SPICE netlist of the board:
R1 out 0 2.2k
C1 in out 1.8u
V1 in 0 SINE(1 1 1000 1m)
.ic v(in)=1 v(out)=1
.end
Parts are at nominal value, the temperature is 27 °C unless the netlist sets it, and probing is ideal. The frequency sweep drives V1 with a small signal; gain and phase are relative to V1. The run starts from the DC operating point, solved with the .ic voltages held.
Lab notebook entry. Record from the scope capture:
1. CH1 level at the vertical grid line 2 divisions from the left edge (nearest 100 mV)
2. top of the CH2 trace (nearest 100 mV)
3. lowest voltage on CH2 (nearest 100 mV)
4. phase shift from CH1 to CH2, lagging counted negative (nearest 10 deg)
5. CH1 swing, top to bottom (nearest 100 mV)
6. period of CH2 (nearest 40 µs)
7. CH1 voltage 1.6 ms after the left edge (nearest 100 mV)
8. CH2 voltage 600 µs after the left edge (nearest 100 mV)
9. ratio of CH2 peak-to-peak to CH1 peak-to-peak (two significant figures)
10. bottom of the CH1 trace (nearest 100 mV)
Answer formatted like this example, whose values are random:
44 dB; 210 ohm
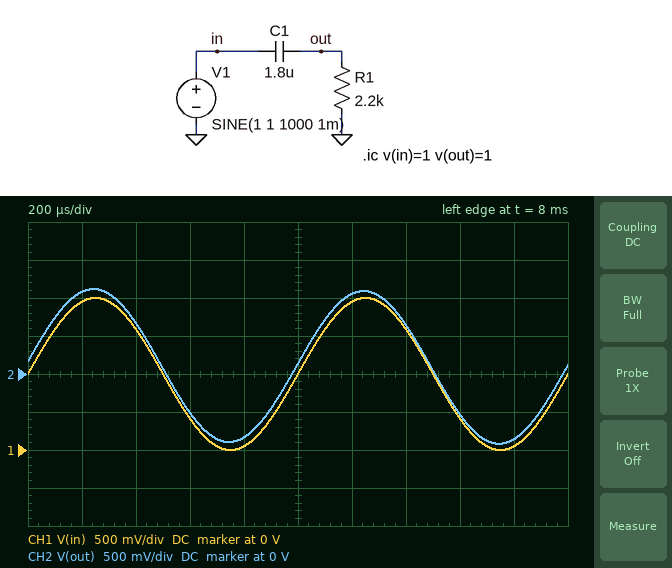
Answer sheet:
1.6 V; 1.1 V; -900 mV; 0 deg; 2.0 V; 1.00 ms; 400 mV; -500 mV; 1.0; 0 V
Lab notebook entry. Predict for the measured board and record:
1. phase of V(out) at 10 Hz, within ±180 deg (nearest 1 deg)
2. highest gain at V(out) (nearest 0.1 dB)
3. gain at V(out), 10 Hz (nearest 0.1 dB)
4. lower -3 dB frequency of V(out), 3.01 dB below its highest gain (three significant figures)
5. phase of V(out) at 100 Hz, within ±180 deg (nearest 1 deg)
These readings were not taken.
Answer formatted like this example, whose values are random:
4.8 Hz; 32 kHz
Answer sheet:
76 deg; 0 dB; -12.3 dB; 40.2 Hz; 22 deg
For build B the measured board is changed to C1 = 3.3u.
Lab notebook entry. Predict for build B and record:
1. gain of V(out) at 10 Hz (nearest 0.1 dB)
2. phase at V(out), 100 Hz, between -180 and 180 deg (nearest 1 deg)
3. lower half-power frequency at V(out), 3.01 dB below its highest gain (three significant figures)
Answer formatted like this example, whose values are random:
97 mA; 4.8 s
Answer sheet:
-7.6 dB; 12 deg; 21.9 Hz
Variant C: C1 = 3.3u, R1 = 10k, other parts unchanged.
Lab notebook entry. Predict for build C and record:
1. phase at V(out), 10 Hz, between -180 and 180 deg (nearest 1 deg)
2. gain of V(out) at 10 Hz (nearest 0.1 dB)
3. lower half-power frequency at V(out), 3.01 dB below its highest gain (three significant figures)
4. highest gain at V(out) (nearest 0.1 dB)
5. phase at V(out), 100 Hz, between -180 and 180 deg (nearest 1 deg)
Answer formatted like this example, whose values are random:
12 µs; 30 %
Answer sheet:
26 deg; -0.9 dB; 4.82 Hz; 0 dB; 3 deg
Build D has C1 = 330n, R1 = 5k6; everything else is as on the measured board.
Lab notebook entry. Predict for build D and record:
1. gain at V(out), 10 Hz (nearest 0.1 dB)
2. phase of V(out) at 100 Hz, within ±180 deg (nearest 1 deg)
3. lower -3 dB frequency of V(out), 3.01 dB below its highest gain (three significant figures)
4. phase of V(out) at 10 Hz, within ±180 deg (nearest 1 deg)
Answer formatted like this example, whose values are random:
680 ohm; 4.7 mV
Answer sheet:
-18.8 dB; 41 deg; 86.1 Hz; 83 deg
